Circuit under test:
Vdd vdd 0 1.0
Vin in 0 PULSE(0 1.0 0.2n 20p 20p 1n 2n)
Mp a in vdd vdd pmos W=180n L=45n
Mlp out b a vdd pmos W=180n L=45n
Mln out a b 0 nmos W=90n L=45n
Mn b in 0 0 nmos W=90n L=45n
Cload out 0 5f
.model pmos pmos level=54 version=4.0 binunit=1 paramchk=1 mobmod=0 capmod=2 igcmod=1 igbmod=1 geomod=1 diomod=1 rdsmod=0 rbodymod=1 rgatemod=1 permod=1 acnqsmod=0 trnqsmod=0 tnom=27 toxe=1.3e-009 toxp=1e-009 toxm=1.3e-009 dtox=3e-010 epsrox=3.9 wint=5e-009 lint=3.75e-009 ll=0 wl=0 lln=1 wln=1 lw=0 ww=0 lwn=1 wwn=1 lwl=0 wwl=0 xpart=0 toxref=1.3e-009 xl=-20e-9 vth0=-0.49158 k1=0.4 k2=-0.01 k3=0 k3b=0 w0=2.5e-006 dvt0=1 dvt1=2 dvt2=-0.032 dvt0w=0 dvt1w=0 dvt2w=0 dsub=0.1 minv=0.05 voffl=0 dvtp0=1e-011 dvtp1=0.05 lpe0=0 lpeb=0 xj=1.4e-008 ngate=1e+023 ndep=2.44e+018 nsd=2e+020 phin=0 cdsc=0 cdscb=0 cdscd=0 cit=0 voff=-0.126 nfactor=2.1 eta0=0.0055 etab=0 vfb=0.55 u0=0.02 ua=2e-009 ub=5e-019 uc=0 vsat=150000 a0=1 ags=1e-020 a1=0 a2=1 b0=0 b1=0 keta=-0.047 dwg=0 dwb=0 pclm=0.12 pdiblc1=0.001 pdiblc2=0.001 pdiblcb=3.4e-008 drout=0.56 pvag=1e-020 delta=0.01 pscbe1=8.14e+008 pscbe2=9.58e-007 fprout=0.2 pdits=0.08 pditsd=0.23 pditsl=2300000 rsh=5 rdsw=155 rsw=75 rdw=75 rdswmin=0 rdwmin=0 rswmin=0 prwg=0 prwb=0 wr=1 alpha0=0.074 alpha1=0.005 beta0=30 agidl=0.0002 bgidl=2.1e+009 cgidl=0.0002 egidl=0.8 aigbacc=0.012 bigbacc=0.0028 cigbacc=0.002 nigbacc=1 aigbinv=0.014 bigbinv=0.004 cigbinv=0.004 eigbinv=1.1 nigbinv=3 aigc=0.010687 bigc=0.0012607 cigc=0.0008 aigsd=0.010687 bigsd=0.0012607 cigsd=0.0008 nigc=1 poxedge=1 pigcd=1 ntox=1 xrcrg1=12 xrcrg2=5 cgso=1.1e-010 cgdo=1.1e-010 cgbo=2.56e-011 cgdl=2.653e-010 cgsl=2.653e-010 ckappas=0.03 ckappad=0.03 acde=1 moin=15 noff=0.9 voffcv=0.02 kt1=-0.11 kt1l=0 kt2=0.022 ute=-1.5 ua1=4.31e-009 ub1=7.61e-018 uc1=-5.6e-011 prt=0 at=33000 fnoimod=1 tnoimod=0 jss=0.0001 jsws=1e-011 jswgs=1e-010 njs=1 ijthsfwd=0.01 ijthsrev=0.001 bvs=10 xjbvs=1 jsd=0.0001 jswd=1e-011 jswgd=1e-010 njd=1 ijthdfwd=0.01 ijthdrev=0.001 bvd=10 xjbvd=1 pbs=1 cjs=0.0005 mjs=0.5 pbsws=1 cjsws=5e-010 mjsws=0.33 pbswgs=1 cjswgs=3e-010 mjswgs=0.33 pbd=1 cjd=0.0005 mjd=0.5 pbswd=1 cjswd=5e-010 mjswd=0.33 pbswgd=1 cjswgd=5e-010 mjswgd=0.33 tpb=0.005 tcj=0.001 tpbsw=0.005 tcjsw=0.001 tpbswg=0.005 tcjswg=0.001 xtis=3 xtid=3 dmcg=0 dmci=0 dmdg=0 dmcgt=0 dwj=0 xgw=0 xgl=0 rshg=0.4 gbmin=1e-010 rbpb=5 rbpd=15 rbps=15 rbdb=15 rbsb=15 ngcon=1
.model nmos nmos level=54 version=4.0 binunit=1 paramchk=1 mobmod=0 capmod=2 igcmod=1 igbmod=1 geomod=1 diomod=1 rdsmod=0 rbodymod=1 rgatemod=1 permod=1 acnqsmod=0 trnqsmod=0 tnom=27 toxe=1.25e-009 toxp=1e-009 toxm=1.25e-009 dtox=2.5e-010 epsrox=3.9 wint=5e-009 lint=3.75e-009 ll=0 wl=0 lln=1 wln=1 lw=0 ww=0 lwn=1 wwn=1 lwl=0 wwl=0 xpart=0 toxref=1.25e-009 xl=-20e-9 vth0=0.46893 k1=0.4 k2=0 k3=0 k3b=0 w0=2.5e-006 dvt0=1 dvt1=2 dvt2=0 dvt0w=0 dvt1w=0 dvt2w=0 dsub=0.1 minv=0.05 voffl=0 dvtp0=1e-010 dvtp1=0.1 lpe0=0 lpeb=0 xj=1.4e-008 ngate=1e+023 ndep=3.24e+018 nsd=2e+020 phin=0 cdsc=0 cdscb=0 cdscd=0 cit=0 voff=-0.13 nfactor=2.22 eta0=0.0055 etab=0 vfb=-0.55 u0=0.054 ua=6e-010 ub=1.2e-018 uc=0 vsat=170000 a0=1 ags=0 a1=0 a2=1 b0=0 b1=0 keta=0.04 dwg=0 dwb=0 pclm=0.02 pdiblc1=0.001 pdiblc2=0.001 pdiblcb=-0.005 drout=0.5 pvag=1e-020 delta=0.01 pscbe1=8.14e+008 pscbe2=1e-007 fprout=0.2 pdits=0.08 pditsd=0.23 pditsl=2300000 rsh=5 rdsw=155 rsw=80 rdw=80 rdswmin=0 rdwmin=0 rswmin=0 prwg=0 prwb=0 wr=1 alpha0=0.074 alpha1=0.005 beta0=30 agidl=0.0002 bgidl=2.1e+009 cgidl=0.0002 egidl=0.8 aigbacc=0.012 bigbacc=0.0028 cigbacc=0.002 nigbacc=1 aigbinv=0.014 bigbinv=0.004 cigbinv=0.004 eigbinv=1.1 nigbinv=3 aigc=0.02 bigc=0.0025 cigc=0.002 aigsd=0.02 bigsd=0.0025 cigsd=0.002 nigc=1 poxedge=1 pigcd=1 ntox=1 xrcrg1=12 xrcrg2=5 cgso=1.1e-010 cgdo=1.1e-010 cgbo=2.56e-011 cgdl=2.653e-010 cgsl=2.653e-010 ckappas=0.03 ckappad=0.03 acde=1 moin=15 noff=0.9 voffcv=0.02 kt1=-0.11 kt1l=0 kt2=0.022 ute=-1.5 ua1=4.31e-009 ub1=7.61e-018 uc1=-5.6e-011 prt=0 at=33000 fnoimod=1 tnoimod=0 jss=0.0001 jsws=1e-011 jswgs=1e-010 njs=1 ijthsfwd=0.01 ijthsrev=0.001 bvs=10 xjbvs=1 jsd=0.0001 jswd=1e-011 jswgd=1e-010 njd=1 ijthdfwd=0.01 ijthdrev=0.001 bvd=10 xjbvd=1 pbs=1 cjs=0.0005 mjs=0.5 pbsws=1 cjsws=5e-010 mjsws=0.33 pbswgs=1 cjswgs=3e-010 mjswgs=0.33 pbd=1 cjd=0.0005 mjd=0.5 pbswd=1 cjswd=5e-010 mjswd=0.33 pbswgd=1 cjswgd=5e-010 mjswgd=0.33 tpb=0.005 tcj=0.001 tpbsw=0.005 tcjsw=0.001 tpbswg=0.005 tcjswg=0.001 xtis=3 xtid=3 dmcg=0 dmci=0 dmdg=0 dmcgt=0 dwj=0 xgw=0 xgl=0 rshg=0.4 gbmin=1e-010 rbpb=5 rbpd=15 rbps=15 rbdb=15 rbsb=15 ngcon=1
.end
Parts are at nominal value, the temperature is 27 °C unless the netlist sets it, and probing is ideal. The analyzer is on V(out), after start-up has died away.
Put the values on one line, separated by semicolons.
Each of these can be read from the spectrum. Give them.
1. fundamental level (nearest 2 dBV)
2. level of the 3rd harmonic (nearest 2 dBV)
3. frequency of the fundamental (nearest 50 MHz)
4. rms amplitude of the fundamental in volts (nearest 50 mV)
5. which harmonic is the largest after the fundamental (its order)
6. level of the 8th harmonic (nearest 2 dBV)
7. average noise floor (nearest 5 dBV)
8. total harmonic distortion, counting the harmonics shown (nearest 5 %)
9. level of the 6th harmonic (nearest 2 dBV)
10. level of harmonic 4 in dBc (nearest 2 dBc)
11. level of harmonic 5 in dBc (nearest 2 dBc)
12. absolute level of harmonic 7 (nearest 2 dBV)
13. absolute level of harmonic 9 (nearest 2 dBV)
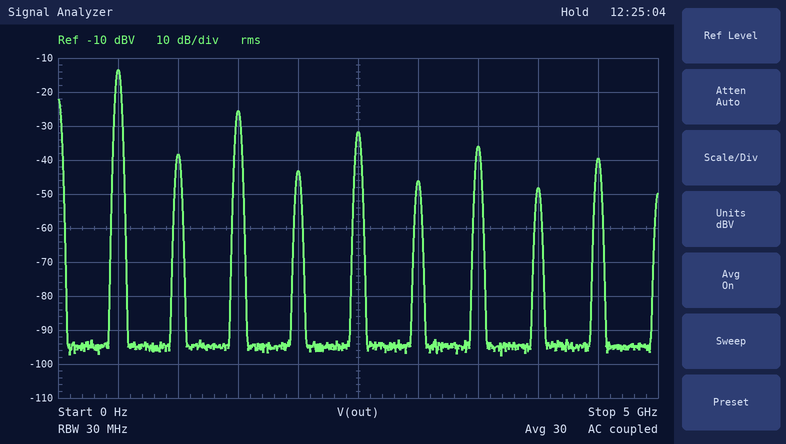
-14 dBV; -26 dBV; 500 MHz; 200 mV; 3; -48 dBV; -95 dBV; 30 %; -46 dBV; -30 dBc; -18 dBc; -36 dBV; -40 dBV
